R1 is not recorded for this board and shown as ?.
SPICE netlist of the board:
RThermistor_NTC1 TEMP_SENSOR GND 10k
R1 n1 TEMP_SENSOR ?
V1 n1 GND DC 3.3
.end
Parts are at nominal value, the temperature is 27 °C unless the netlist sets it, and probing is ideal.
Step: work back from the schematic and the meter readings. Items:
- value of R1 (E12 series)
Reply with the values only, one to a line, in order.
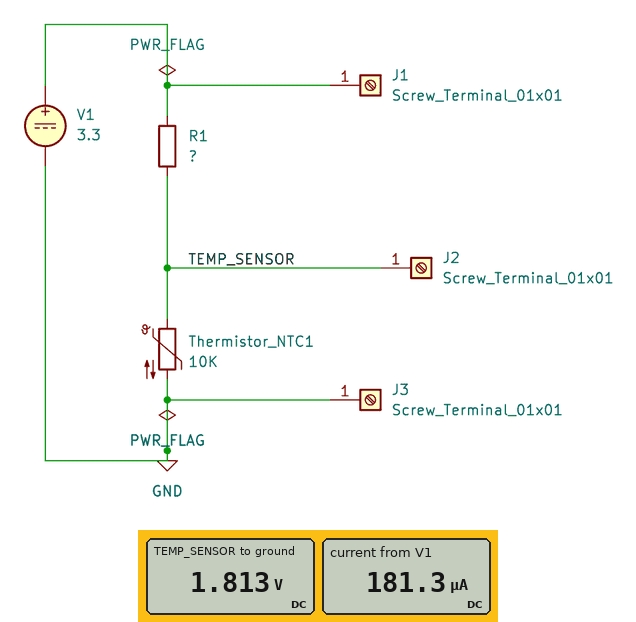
8.2 kΩ
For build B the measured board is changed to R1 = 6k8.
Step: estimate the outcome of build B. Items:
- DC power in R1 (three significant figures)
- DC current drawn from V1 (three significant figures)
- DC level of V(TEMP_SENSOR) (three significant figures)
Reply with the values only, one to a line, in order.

262 µW
196 µA
1.96 V
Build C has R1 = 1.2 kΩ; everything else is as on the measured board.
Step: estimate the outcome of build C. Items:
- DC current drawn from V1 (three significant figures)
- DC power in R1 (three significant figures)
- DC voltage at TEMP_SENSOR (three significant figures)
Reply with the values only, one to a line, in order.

295 µA
104 µW
2.95 V
